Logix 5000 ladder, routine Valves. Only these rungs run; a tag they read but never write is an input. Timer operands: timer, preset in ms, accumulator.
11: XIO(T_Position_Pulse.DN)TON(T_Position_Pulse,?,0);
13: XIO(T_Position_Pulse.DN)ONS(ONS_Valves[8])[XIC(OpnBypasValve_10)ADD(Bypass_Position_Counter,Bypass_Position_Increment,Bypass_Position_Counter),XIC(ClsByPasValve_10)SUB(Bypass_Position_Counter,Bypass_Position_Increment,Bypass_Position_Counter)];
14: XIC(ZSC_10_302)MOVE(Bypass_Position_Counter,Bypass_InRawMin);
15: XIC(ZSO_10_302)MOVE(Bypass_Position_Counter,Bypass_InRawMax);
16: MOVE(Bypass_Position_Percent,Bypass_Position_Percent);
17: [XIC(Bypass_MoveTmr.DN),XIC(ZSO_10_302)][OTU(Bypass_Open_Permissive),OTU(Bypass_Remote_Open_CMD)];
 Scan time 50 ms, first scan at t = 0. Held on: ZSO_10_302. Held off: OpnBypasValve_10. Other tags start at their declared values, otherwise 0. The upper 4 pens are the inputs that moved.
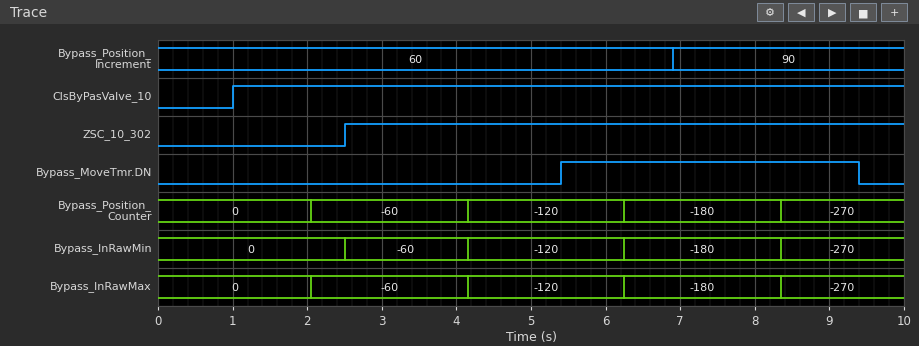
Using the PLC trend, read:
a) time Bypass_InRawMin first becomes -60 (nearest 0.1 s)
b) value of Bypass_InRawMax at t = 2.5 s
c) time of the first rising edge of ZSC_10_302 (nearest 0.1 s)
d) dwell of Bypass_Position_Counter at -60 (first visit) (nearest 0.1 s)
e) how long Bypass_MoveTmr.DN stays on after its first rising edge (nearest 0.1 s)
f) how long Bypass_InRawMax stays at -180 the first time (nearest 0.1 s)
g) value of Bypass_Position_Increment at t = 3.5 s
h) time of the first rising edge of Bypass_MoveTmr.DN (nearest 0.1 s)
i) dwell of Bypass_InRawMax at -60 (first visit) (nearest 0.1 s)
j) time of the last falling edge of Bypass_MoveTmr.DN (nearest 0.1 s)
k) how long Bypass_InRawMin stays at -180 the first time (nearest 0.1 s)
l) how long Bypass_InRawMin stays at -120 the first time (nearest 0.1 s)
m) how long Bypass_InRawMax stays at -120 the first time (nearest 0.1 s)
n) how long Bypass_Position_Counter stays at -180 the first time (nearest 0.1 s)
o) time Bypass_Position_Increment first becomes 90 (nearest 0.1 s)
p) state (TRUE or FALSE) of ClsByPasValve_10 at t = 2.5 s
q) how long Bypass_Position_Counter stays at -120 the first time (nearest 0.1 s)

2.5 s
-60
2.5 s
2.1 s
4.0 s
2.1 s
60
5.4 s
2.1 s
9.4 s
2.1 s
2.1 s
2.1 s
2.1 s
6.9 s
TRUE
2.1 s
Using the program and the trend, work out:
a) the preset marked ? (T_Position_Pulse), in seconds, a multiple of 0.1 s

2.0 s
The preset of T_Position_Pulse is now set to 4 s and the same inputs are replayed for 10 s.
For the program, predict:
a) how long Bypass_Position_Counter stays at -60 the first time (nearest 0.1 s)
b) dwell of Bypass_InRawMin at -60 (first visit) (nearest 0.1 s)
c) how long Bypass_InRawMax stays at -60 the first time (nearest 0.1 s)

4.1 s
4.1 s
4.1 s
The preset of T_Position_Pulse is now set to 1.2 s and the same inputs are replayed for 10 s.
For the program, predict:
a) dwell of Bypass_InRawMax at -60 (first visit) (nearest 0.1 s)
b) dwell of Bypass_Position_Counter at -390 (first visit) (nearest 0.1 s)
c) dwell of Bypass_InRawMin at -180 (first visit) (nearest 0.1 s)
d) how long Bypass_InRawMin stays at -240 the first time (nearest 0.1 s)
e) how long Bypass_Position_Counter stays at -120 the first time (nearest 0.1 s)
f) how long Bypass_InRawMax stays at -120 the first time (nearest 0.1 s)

1.3 s
1.3 s
1.3 s
1.3 s
1.3 s
1.3 s
